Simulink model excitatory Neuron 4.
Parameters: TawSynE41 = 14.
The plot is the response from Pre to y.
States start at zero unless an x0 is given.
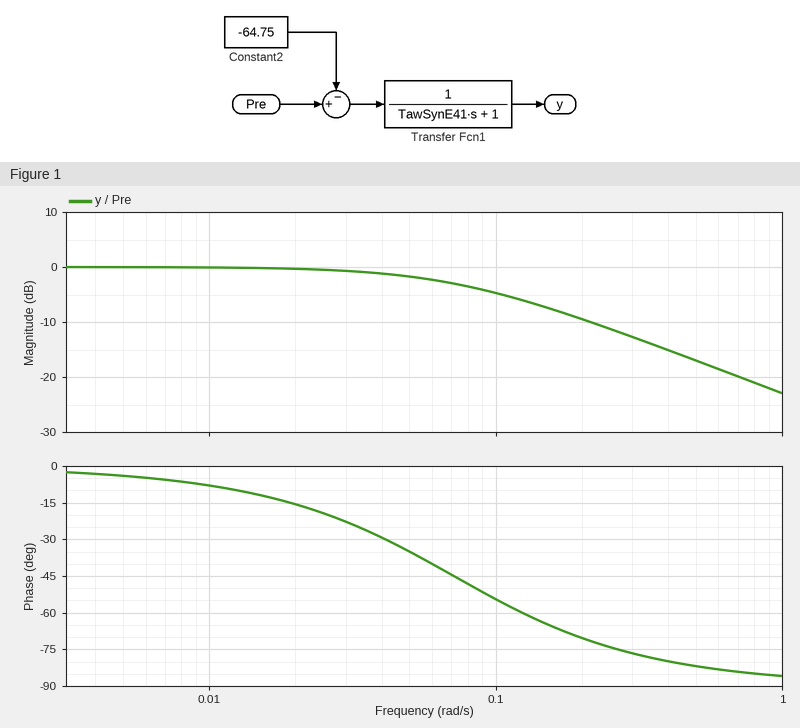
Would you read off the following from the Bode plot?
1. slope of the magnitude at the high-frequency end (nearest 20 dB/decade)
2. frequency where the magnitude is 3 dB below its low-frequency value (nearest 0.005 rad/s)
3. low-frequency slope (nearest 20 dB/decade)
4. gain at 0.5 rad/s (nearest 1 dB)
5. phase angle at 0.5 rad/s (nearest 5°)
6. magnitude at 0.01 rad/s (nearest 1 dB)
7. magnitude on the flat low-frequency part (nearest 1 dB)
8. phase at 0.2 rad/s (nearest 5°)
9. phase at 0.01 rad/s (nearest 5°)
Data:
-20 dB/decade
0.070 rad/s
0 dB/decade
-17 dB
-80°
0 dB
0 dB
-70°
-10°
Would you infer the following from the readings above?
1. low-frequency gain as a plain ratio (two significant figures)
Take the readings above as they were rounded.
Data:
1.0
